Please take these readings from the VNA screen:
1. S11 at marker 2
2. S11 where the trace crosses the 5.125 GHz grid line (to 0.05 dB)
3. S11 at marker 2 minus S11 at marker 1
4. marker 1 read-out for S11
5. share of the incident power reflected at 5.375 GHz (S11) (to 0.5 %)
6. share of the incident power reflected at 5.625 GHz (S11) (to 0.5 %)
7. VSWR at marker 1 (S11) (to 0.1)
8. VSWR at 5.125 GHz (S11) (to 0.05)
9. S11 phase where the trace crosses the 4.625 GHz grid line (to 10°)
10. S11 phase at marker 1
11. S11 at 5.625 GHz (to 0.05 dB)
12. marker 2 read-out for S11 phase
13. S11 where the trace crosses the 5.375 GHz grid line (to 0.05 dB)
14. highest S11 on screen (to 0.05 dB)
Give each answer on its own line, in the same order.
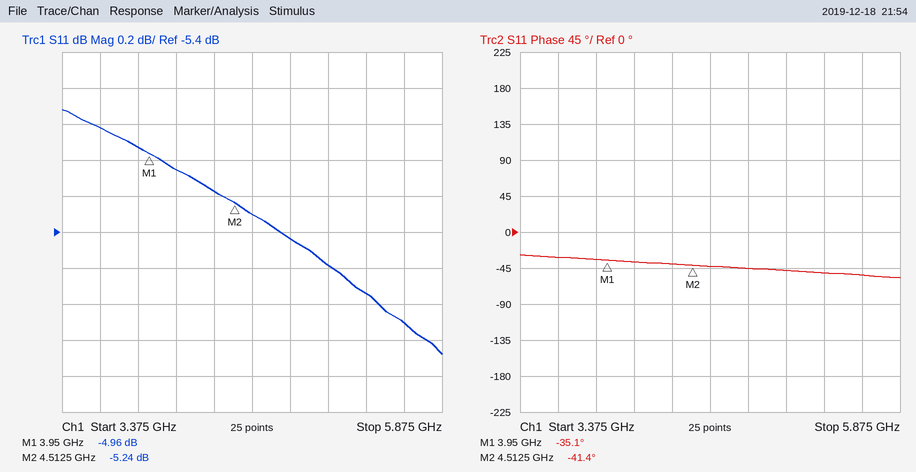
-5.24 dB
-5.60 dB
-0.28 dB
-4.96 dB
26.5 %
25.5 %
3.6
3.20
-40°
-35.1°
-5.90 dB
-41.4°
-5.75 dB
-4.70 dB
